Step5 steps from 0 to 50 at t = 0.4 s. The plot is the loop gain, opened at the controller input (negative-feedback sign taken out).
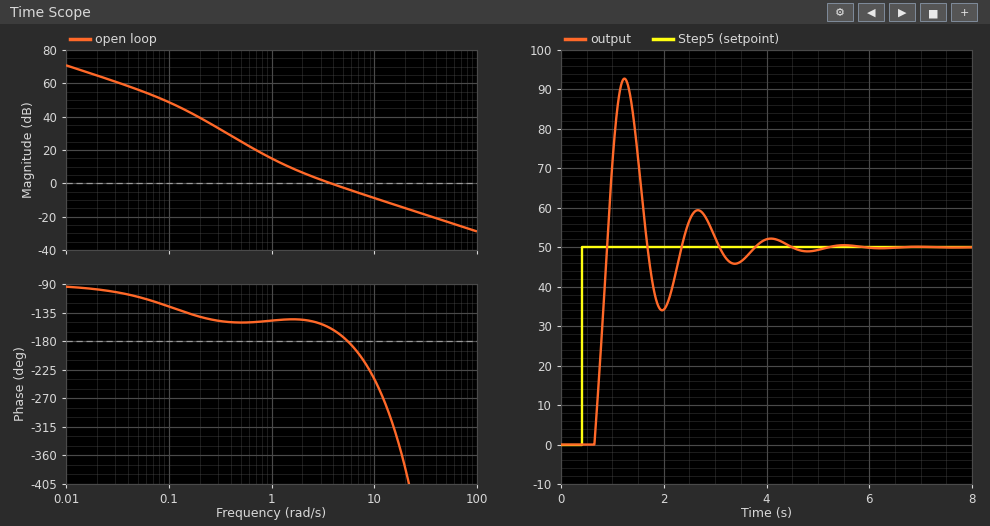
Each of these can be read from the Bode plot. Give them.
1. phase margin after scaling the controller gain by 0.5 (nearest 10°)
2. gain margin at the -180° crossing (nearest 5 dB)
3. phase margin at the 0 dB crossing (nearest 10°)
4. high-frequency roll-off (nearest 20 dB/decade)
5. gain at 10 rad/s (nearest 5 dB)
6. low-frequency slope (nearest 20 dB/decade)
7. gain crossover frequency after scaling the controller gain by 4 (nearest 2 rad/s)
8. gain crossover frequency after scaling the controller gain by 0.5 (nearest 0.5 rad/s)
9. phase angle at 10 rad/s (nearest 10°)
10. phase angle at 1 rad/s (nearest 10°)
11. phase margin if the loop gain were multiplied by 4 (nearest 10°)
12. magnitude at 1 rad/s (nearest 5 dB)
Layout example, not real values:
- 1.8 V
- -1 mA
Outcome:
- 30°
- 5 dB
- 20°
- -20 dB/decade
- -10 dB
- -20 dB/decade
- 14 rad/s
- 2.0 rad/s
- -240°
- -150°
- -120°
- 15 dB
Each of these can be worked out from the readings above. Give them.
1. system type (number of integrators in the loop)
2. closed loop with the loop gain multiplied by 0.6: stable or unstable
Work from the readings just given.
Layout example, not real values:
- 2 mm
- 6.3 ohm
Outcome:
- 1
- stable
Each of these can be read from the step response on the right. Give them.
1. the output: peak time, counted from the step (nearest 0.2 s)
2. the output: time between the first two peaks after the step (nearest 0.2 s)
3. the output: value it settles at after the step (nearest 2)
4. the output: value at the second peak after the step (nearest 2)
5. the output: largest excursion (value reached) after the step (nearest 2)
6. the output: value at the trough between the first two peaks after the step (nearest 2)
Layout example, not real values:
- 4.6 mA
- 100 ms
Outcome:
- 0.8 s
- 1.4 s
- 50
- 60
- 92
- 34
